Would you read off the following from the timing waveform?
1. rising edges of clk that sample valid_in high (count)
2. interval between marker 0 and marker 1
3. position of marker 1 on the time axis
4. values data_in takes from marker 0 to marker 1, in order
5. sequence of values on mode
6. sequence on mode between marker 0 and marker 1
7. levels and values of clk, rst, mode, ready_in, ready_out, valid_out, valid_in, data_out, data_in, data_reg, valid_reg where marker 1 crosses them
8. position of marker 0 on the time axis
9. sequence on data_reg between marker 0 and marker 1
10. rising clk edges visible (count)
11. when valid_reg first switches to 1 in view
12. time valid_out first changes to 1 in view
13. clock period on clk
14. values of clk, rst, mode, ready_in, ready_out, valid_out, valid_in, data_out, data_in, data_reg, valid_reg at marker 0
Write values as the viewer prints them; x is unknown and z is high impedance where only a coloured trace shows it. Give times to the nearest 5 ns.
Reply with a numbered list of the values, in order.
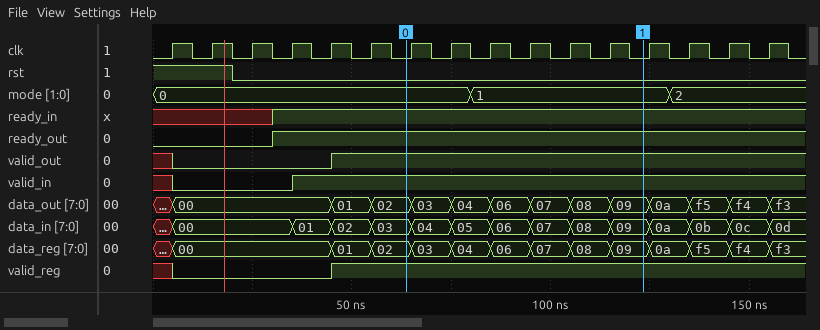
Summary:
1. 12
2. 60 ns
3. 125 ns
4. 03, 04, 05, 06, 07, 08, 09
5. 0, 1, 2
6. 0, 1
7. clk=0, rst=0, mode=1, ready_in=1, ready_out=1, valid_out=1, valid_in=1, data_out=09, data_in=09, data_reg=09, valid_reg=1
8. 65 ns
9. 02, 03, 04, 06, 07, 08, 09
10. 16
11. 45 ns
12. 45 ns
13. 10 ns
14. clk=0, rst=0, mode=0, ready_in=1, ready_out=1, valid_out=1, valid_in=1, data_out=02, data_in=03, data_reg=02, valid_reg=1
